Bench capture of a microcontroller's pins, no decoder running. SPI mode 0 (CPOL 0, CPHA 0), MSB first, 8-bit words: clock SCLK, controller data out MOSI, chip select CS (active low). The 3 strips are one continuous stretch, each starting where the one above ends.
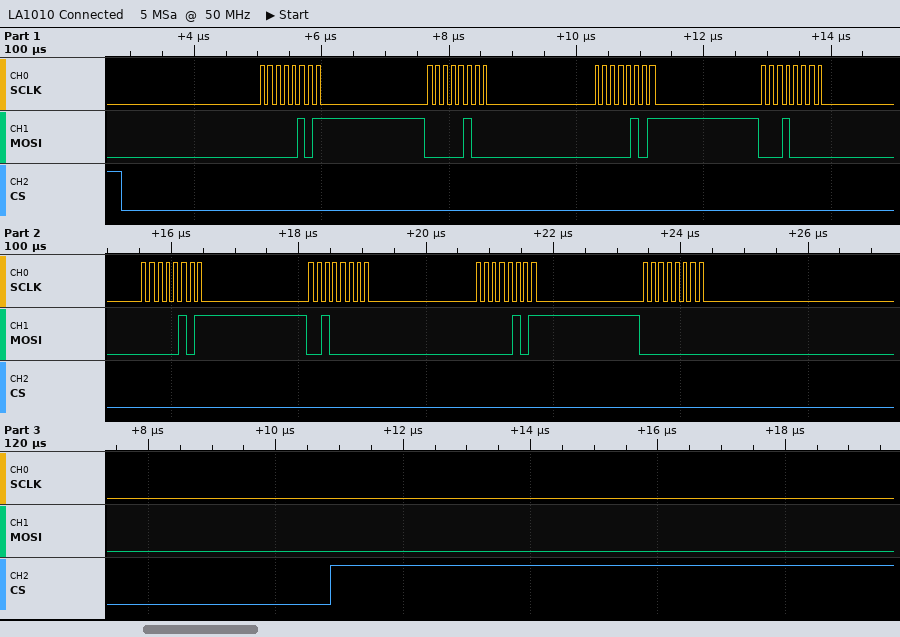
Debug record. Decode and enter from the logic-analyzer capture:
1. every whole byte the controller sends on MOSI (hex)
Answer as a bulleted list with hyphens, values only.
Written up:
- 05 04 05 10 05 20 05 00
